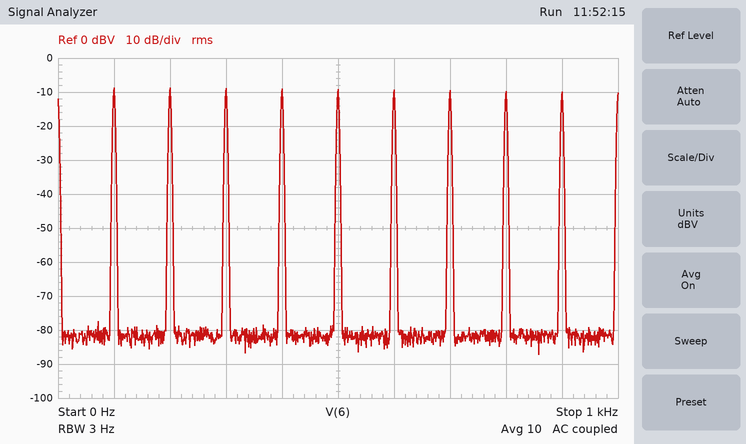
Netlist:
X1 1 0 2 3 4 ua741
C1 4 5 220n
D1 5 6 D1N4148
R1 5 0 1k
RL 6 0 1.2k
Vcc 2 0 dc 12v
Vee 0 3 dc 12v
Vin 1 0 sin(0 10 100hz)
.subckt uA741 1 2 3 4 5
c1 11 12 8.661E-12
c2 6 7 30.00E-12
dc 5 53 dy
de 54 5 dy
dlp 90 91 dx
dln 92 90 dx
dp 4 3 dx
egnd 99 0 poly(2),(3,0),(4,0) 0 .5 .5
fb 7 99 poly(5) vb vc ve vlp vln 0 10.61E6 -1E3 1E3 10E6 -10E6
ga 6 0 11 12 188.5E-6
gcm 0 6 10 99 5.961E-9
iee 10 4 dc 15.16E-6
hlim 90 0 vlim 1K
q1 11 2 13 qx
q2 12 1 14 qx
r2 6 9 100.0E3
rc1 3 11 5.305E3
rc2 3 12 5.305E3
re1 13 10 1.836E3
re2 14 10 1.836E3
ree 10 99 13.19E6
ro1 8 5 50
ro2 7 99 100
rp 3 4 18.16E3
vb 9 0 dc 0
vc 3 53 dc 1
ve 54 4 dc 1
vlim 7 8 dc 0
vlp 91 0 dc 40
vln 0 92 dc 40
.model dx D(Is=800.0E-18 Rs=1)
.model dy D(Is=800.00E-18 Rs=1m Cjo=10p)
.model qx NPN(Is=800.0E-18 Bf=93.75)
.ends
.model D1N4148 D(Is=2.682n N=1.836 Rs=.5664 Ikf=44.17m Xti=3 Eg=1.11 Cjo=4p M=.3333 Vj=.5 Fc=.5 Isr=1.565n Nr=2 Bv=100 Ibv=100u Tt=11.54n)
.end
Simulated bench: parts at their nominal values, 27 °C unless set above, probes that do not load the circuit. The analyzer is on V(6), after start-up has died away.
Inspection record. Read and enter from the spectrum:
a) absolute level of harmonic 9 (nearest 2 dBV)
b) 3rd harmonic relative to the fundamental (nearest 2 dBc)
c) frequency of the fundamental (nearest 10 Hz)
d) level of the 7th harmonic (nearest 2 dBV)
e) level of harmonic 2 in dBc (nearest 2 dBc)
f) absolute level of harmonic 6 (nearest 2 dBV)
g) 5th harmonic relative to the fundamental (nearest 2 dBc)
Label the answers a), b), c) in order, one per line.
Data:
a) -10 dBV
b) 0 dBc
c) 100 Hz
d) -10 dBV
e) 0 dBc
f) -10 dBV
g) 0 dBc
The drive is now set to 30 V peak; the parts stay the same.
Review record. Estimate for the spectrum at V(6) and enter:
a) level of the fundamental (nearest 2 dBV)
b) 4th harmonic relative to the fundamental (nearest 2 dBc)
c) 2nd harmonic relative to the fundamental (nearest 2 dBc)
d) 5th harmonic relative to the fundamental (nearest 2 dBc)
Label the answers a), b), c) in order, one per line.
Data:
a) -16 dBV
b) 10 dBc
c) 12 dBc
d) 12 dBc
